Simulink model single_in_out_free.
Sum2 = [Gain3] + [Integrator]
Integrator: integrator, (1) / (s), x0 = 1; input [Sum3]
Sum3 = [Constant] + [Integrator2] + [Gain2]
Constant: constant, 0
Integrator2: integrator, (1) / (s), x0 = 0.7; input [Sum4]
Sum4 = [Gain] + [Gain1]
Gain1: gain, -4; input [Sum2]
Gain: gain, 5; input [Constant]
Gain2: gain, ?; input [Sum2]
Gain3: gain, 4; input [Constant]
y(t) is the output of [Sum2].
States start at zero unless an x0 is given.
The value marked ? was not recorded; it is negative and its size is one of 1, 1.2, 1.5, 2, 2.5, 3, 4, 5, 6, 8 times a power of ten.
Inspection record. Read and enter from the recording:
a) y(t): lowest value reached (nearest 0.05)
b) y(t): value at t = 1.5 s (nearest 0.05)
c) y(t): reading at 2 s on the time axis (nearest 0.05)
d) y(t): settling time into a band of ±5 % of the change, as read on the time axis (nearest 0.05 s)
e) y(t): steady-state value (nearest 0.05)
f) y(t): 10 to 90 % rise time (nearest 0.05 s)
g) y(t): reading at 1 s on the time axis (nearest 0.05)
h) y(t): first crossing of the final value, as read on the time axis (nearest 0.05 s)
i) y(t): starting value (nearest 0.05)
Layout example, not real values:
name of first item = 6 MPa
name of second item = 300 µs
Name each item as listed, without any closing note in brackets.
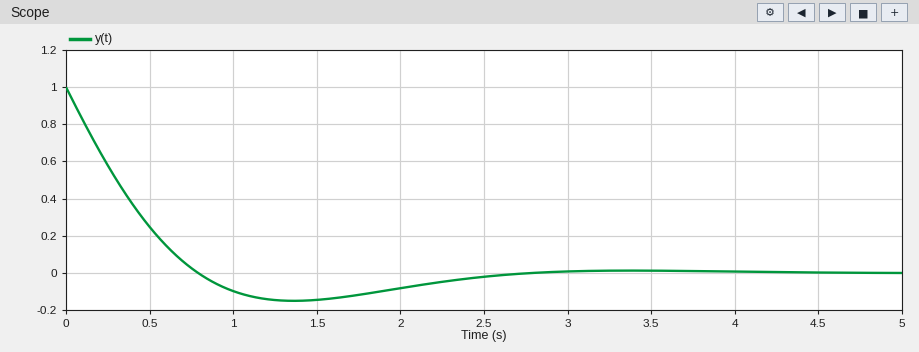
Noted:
y(t): lowest value reached = -0.15
y(t): value at t = 1.5 s = -0.15
y(t): reading at 2 s on the time axis = -0.10
y(t): settling time into a band of ±5 % of the change, as read on the time axis = 2.25 s
y(t): steady-state value = 0.00
y(t): 10 to 90 % rise time = 0.60 s
y(t): reading at 1 s on the time axis = -0.10
y(t): first crossing of the final value, as read on the time axis = 0.80 s
y(t): starting value = 1.00
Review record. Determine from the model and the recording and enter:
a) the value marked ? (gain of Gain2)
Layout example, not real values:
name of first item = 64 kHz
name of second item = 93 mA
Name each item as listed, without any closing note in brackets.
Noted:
the value marked ? = -2.5
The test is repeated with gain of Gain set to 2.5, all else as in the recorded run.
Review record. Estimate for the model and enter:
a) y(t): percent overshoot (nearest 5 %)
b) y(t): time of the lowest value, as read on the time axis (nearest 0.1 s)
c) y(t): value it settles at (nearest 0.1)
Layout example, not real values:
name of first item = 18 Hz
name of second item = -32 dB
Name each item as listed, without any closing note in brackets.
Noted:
y(t): percent overshoot = 15 %
y(t): time of the lowest value, as read on the time axis = 1.4 s
y(t): value it settles at = 0.0
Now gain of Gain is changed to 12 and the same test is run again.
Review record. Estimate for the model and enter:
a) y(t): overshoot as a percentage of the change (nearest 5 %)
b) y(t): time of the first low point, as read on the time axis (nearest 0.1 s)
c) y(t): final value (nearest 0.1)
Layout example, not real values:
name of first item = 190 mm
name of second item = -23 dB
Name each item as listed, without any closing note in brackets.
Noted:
y(t): overshoot as a percentage of the change = 15 %
y(t): time of the first low point, as read on the time axis = 1.4 s
y(t): final value = 0.0
